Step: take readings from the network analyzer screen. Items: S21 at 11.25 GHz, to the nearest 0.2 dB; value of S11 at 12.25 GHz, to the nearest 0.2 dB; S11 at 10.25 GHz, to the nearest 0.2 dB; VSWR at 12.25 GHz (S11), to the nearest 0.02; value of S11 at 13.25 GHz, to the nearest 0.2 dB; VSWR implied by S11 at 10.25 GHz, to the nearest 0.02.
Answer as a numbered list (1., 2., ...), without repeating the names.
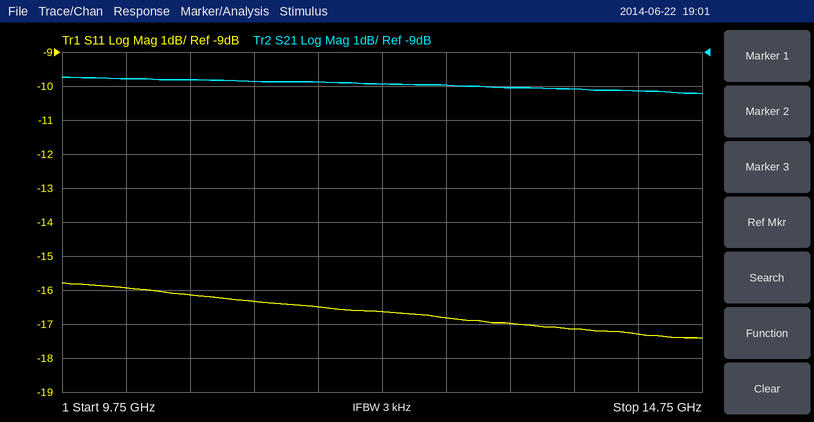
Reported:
1. -9.8 dB
2. -16.6 dB
3. -16.0 dB
4. 1.34
5. -17.0 dB
6. 1.38
